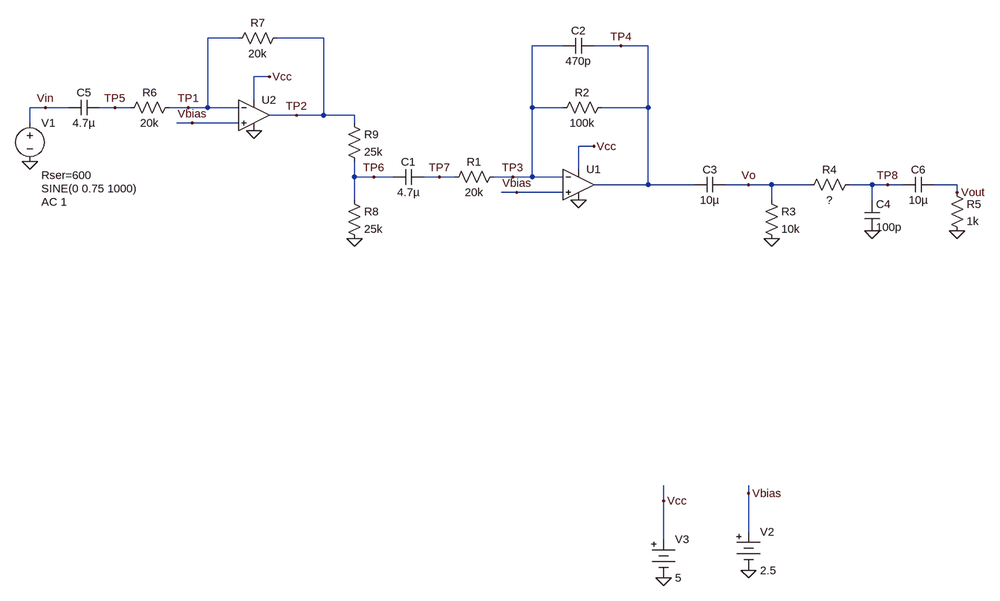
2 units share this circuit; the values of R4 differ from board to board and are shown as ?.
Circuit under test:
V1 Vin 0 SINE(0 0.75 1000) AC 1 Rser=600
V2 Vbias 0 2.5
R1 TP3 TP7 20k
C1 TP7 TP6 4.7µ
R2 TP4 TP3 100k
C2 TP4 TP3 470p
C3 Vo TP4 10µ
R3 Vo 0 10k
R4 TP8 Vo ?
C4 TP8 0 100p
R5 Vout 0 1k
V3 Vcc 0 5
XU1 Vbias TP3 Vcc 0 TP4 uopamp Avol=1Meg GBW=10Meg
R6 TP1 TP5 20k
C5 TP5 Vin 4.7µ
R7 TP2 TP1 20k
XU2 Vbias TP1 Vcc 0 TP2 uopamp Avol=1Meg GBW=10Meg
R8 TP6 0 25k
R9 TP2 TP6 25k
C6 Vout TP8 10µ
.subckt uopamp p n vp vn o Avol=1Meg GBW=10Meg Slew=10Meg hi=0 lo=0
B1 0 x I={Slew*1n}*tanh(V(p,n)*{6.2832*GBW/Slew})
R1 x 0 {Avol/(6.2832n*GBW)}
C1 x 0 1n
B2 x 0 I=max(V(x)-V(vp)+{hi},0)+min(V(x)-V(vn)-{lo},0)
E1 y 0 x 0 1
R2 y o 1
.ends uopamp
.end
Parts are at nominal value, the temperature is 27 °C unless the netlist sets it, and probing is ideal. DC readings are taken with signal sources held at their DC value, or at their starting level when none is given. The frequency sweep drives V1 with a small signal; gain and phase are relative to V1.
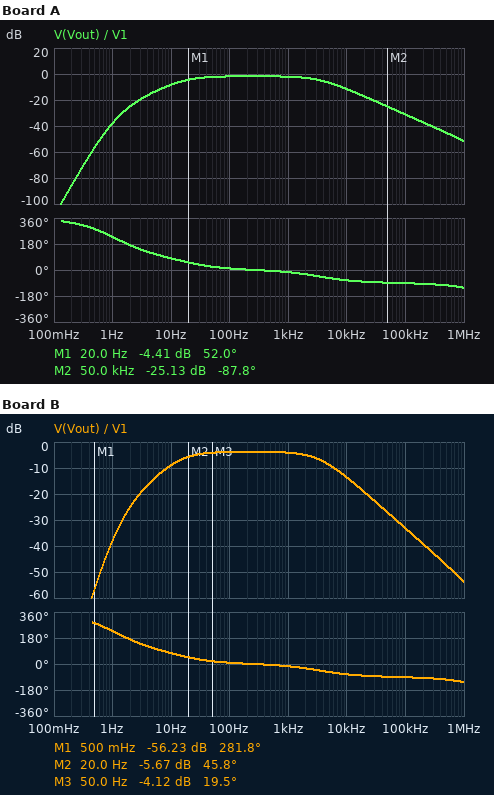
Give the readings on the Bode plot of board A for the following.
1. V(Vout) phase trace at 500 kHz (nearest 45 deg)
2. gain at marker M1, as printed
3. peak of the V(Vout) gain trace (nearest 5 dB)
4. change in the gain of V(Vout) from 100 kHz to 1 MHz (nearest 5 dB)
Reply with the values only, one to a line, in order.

-90 deg
-4.41 dB
0 dB
-20 dB
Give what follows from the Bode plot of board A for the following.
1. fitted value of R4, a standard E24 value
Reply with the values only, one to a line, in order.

820 Ω
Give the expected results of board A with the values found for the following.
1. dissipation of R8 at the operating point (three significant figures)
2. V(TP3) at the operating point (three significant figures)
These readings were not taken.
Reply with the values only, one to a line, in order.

62.5 µW
2.50 V
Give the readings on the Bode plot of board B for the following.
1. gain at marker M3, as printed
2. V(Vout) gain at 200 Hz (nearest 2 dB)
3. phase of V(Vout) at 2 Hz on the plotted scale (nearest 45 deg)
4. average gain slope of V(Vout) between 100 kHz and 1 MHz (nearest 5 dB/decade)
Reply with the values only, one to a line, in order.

-4.12 dB
-4 dB
180 deg
-20 dB/decade
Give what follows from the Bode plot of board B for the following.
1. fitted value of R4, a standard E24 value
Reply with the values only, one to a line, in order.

1.3 kΩ
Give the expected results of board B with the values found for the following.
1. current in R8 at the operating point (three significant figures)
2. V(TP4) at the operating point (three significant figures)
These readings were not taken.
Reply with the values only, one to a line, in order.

50.0 µA
2.50 V
